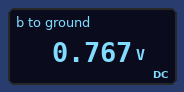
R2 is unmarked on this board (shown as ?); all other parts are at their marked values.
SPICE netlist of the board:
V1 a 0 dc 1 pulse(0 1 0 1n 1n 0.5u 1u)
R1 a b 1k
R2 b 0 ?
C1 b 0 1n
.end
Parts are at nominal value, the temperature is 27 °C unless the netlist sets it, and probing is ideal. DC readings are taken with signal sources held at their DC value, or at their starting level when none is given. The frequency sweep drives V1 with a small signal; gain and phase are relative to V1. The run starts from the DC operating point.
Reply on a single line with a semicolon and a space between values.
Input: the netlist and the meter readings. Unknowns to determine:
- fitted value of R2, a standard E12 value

3.3 kΩ
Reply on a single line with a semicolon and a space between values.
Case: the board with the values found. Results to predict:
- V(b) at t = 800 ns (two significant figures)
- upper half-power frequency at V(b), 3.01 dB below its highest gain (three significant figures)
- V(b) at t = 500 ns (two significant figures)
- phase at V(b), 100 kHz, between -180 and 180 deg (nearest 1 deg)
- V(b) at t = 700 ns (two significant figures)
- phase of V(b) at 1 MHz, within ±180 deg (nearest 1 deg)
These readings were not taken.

250 mV; 207 kHz; 370 mV; -26 deg; 280 mV; -78 deg
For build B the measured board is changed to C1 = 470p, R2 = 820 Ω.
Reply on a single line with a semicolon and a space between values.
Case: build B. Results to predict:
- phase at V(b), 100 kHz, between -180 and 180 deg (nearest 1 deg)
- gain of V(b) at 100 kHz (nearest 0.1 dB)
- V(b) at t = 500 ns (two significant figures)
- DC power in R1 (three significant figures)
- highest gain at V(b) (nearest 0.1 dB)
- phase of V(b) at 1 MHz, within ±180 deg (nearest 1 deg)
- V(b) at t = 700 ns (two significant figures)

-8 deg; -7.0 dB; 410 mV; 302 µW; -6.9 dB; -53 deg; 160 mV
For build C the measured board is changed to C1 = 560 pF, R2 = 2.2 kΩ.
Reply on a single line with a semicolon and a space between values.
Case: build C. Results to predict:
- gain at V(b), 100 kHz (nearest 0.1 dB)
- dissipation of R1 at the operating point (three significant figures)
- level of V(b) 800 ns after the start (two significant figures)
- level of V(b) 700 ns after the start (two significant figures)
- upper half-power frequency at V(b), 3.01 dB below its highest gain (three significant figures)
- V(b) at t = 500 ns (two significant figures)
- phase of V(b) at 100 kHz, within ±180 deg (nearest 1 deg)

-3.5 dB; 97.7 µW; 230 mV; 300 mV; 413 kHz; 500 mV; -14 deg
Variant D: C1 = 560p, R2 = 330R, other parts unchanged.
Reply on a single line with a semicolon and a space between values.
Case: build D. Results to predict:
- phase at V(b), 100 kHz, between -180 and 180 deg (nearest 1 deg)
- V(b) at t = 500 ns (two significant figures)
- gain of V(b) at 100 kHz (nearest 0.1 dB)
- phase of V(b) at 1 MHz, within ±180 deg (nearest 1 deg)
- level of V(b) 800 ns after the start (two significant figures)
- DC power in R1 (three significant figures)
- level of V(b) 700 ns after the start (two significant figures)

-5 deg; 240 mV; -12.1 dB; -41 deg; 28 mV; 565 µW; 58 mV
